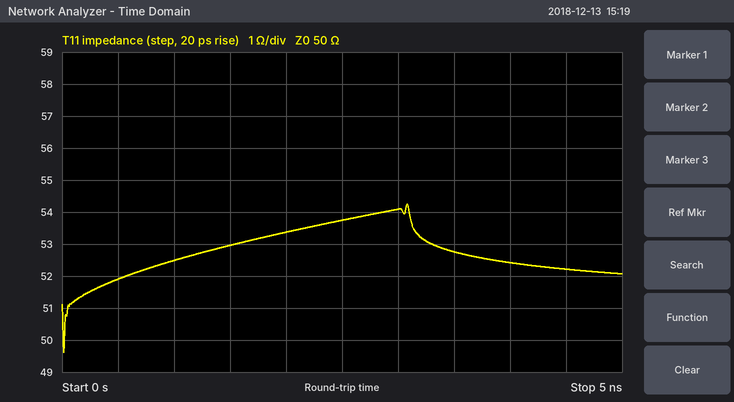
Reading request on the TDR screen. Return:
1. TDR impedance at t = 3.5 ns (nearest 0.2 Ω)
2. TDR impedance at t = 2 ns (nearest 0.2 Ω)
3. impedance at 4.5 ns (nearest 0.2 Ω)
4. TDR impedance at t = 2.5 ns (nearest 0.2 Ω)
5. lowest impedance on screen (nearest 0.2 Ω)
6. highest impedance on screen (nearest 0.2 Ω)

52.8 Ω
53.4 Ω
52.2 Ω
53.8 Ω
49.6 Ω
54.2 Ω
